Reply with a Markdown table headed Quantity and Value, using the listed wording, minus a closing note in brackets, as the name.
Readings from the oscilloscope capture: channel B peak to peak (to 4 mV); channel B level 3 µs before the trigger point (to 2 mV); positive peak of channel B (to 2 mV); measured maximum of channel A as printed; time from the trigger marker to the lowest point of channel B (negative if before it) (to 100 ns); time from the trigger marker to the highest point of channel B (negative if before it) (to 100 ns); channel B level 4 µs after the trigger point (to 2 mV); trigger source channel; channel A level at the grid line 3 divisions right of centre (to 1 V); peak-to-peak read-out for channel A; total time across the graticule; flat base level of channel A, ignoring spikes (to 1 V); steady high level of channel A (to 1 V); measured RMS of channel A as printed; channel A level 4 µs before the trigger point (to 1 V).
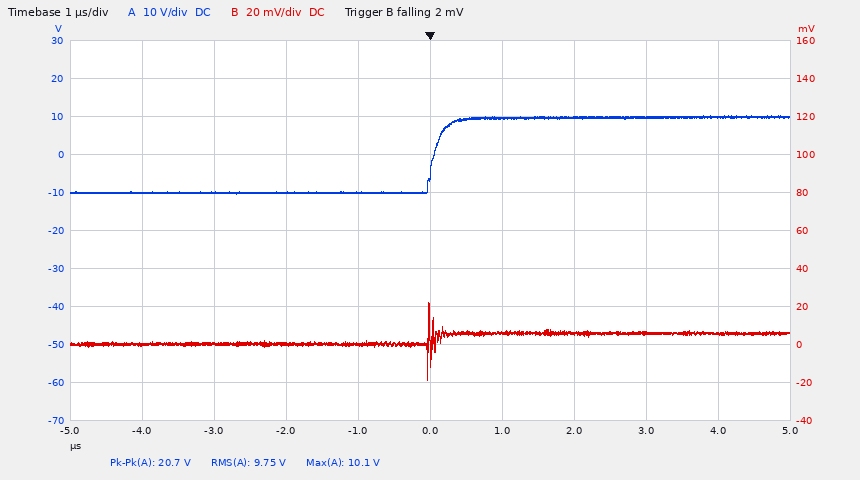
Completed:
| Quantity | Value |
|---|---|
| channel B peak to peak | 40 mV |
| channel B level 3 µs before the trigger point | 0 mV |
| positive peak of channel B | 22 mV |
| measured maximum of channel A as printed | 10.1 V |
| time from the trigger marker to the lowest point of channel B (negative if before it) | 0.0 µs |
| time from the trigger marker to the highest point of channel B (negative if before it) | 0.0 µs |
| channel B level 4 µs after the trigger point | 6 mV |
| trigger source channel | channel B |
| channel A level at the grid line 3 divisions right of centre | 10 V |
| peak-to-peak read-out for channel A | 20.7 V |
| total time across the graticule | 10 µs |
| flat base level of channel A, ignoring spikes | -10 V |
| steady high level of channel A | 10 V |
| measured RMS of channel A as printed | 9.75 V |
| channel A level 4 µs before the trigger point | -10 V |
